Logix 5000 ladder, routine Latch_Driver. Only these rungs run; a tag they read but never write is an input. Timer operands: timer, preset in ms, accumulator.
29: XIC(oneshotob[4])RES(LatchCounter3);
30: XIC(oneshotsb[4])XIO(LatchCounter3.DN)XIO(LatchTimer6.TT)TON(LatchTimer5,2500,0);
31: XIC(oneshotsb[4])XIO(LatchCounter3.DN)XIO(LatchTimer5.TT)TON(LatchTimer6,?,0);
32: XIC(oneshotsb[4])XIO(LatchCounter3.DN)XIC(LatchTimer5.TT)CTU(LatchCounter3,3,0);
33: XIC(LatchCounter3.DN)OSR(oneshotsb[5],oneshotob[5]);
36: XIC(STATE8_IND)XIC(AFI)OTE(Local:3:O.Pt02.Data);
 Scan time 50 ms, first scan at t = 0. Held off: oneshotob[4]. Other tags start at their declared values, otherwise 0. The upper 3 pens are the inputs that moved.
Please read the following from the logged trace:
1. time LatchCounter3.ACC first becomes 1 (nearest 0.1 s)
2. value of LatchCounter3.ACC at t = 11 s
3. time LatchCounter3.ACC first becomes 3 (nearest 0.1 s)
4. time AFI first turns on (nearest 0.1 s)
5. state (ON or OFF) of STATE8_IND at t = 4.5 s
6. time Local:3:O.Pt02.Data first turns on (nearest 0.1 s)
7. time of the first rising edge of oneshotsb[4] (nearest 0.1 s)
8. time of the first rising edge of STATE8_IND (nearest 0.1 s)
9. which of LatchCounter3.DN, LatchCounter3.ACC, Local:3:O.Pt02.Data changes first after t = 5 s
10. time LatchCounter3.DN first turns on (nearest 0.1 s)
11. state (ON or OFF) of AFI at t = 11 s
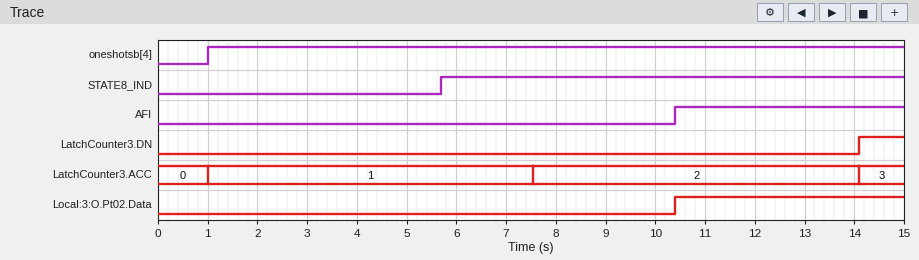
1.0 s
2
14.1 s
10.4 s
OFF
10.4 s
1.0 s
5.7 s
LatchCounter3.ACC
14.1 s
ON
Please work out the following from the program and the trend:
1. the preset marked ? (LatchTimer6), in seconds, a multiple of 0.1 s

4.0 s
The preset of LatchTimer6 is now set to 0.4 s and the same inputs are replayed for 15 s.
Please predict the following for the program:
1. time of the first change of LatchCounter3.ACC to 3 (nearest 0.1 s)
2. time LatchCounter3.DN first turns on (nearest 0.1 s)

6.9 s
6.9 s
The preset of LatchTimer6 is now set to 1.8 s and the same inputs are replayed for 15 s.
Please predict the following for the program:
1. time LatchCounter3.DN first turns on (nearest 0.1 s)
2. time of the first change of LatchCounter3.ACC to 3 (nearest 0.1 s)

9.7 s
9.7 s
